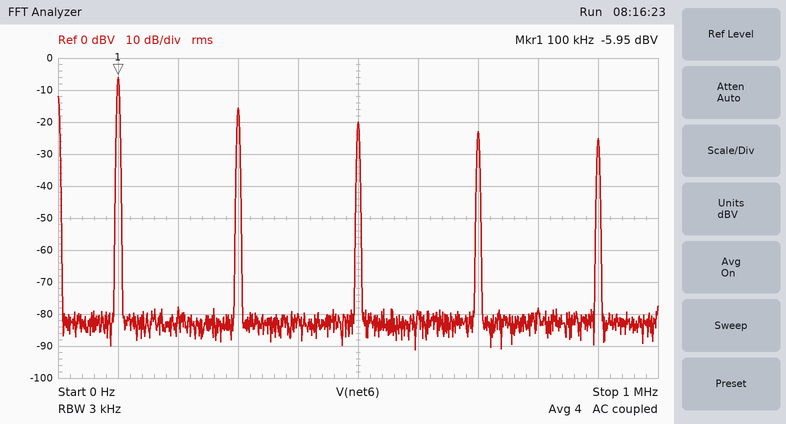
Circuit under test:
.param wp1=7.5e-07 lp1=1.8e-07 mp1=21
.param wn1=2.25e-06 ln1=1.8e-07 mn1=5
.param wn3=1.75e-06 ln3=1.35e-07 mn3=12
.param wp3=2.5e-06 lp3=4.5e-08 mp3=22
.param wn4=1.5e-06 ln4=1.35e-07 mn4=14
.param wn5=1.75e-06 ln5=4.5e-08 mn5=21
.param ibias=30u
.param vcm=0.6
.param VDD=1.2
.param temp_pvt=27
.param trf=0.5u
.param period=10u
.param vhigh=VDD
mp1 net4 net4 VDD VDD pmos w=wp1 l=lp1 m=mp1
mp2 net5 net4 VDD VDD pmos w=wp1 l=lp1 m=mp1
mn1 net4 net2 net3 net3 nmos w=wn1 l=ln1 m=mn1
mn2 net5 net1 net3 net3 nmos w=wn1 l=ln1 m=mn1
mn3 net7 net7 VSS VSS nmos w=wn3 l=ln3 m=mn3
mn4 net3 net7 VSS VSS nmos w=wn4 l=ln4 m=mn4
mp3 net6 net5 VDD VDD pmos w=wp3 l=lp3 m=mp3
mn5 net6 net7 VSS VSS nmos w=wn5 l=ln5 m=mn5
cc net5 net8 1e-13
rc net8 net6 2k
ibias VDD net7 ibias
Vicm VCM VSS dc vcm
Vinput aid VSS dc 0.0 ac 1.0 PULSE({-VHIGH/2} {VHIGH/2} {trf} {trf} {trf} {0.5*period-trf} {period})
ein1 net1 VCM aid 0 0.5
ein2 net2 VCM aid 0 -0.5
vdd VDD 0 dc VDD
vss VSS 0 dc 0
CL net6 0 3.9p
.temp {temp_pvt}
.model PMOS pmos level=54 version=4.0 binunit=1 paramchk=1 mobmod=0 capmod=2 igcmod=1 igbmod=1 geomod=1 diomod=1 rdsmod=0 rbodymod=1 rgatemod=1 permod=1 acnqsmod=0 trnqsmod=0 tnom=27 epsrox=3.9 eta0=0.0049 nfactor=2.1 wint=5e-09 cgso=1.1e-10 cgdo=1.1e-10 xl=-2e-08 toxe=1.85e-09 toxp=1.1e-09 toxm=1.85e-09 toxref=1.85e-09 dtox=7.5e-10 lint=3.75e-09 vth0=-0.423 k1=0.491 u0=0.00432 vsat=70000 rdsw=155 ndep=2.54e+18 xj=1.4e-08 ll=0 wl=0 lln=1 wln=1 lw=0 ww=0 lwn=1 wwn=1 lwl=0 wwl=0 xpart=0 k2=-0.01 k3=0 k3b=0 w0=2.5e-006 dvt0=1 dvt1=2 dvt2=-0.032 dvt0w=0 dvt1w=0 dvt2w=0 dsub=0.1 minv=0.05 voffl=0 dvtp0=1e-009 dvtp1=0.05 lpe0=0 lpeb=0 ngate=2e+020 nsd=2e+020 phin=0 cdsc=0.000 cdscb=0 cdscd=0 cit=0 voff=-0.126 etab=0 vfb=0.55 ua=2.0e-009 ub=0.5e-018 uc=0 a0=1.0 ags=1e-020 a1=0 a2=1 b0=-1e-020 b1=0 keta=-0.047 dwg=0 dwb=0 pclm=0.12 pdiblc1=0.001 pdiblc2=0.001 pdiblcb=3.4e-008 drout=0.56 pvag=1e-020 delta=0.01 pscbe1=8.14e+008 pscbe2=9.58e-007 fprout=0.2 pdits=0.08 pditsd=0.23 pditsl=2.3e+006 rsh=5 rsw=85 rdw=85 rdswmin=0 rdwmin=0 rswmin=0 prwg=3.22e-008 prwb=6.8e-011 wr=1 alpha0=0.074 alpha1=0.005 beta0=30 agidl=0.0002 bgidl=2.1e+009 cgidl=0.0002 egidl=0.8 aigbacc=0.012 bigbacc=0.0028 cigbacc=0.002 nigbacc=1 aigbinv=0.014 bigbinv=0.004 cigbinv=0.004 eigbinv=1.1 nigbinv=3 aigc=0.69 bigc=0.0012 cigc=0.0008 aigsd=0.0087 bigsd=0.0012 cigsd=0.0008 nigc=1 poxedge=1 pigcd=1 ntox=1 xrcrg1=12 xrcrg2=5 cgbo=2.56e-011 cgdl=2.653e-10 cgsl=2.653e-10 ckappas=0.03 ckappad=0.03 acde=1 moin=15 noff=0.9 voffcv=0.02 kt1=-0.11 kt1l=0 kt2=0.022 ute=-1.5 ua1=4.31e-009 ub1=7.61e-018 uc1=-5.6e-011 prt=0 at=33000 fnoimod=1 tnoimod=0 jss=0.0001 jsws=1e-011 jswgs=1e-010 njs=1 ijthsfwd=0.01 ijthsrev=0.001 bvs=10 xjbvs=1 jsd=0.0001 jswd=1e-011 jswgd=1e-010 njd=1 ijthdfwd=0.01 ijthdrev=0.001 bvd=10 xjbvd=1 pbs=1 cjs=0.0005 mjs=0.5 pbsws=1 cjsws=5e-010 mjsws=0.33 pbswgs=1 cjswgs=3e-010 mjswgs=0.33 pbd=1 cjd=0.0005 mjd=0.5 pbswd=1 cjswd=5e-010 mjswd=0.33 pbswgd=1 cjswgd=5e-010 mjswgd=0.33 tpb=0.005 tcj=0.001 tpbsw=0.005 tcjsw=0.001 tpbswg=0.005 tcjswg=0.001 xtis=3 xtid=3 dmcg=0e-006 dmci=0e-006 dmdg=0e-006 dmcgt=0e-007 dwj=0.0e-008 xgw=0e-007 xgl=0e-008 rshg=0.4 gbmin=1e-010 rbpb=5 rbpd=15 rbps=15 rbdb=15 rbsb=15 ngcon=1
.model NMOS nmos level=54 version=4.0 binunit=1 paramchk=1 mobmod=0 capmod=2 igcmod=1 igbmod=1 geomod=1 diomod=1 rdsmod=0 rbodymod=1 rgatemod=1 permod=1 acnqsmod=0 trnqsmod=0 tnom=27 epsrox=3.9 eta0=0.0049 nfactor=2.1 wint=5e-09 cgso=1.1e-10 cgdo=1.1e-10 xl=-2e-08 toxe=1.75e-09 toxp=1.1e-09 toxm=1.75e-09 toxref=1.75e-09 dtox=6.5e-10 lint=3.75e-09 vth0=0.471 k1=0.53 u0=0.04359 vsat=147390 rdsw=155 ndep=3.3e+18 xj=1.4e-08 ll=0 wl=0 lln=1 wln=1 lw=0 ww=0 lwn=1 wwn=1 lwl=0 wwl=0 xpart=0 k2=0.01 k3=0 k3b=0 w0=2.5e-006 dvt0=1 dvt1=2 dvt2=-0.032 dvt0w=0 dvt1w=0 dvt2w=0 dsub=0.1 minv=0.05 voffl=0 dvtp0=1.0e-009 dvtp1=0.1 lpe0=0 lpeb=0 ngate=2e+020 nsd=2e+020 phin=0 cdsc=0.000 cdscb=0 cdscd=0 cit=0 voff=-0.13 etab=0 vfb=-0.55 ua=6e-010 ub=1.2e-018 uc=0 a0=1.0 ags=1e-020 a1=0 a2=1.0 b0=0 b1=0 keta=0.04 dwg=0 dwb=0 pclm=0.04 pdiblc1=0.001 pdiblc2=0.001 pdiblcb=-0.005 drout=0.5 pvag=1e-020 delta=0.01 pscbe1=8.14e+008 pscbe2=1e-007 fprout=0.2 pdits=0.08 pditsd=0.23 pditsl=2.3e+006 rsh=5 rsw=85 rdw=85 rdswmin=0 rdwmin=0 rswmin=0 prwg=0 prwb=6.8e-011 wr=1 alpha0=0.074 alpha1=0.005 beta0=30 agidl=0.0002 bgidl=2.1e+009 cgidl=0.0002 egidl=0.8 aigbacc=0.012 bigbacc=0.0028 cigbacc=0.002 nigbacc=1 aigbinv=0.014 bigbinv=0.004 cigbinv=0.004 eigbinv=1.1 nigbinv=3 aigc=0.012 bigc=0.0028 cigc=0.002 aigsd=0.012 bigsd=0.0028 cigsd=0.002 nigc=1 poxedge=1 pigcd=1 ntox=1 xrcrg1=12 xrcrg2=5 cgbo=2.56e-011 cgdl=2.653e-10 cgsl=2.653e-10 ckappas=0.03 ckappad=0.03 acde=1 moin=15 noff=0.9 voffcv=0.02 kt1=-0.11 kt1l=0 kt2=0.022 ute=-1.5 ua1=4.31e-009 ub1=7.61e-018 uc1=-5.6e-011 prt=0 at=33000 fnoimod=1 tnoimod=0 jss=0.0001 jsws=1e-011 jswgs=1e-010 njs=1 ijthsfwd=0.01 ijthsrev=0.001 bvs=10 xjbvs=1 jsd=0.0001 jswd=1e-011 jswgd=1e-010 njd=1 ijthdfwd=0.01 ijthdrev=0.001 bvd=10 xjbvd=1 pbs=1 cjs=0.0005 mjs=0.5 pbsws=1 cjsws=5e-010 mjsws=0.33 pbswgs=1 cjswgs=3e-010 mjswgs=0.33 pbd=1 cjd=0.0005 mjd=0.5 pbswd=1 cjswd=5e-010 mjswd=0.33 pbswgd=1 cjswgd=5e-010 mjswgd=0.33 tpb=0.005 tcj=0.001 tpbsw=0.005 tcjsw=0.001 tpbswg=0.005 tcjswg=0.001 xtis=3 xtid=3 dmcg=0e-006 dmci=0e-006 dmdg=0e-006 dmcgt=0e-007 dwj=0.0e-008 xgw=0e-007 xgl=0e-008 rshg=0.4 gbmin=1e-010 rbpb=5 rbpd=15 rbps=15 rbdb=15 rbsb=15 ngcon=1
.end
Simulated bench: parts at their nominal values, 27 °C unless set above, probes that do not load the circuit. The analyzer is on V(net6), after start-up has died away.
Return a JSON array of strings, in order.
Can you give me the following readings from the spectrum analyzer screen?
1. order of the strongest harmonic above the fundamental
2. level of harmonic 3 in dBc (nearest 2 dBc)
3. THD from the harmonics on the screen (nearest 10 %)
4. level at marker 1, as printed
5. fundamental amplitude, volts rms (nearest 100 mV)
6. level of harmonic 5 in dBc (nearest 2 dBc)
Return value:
["3", "-10 dBc", "40 %", "-5.95 dBV", "500 mV", "-14 dBc"]
